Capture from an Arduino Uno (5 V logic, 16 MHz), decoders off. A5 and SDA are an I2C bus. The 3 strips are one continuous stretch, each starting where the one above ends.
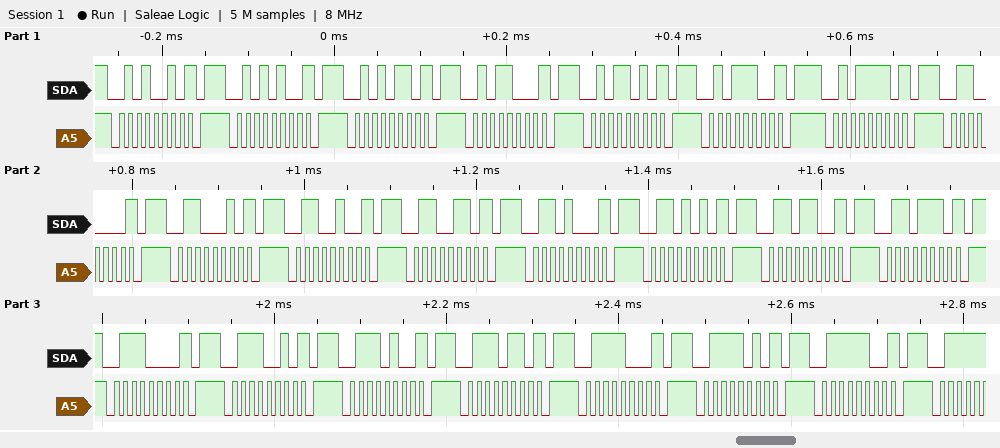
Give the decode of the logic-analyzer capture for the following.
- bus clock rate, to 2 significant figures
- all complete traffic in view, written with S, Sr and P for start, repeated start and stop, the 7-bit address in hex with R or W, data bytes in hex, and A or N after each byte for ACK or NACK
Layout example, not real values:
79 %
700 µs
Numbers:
100 kHz
S 29W N P S 2AW N P S 2BW N P S 2CW N P S 2DW N P S 2EW N P S 2FW N P S 30W N P S 31W N P S 32W N P S 33W N P S 34W N P S 35W N P S 36W N P S 37W N P S 38W N P S 39W N P S 3AW N P S 3BW N P S 3CW N P S 3DW N P S 3EW N P
